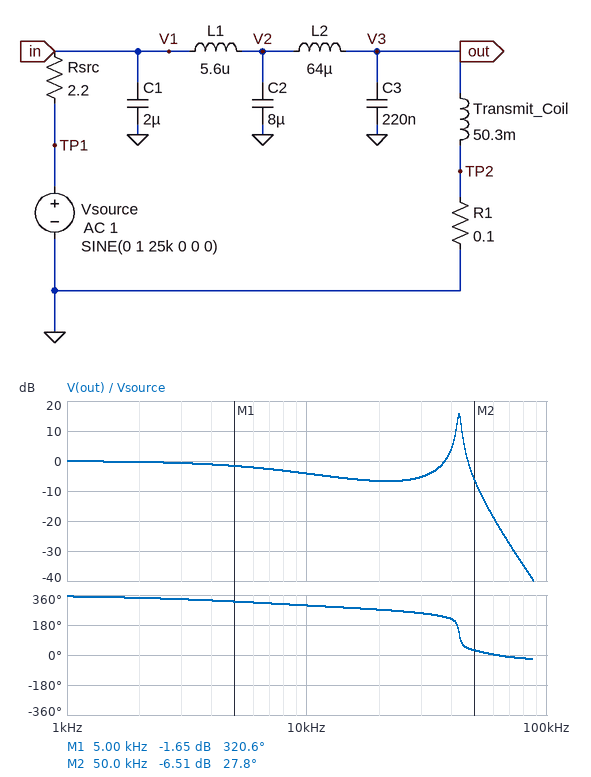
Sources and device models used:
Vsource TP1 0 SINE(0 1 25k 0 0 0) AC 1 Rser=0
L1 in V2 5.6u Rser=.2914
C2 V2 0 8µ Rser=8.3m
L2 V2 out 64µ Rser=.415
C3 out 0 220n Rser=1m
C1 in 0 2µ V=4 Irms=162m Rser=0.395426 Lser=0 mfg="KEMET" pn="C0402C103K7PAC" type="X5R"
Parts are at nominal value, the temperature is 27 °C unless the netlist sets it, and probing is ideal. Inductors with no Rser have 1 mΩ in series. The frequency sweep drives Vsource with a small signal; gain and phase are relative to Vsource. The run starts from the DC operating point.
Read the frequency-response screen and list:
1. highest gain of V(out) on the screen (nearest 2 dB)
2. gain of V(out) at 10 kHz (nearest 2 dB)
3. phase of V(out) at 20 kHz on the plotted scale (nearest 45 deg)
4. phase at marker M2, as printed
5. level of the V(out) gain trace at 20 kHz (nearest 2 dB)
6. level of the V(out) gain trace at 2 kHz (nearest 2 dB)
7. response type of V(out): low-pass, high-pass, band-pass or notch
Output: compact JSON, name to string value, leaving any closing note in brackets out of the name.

{"highest gain of V(out) on the screen": "16 dB", "gain of V(out) at 10 kHz": "-4 dB", "phase of V(out) at 20 kHz on the plotted scale": "270 deg", "phase at marker M2, as printed": "27.8 deg", "level of the V(out) gain trace at 20 kHz": "-6 dB", "level of the V(out) gain trace at 2 kHz": "0 dB", "response type of V(out): low-pass, high-pass, band-pass or notch": "band-pass"}
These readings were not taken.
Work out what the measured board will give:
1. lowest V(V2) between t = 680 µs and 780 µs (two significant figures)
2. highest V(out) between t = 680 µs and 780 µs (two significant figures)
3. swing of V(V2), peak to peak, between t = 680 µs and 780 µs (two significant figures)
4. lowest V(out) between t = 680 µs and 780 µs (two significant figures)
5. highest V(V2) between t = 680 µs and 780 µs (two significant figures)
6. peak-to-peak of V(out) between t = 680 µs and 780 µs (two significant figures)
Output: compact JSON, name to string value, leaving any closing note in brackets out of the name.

{"lowest V(V2) between t = 680 µs and 780 µs": "-310 mV", "highest V(out) between t = 680 µs and 780 µs": "480 mV", "swing of V(V2), peak to peak, between t = 680 µs and 780 µs": "620 mV", "lowest V(out) between t = 680 µs and 780 µs": "-480 mV", "highest V(V2) between t = 680 µs and 780 µs": "310 mV", "peak-to-peak of V(out) between t = 680 µs and 780 µs": "960 mV"}
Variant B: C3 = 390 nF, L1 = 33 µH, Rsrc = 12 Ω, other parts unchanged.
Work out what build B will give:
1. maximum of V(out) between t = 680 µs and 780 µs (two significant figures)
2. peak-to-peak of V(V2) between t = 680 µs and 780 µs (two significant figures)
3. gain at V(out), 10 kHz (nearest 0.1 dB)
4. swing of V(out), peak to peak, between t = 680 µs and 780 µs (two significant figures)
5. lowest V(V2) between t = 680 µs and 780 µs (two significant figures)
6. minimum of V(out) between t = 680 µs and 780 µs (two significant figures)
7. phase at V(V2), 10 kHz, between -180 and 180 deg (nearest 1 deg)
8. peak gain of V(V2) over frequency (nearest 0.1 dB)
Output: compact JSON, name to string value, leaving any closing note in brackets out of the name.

{"maximum of V(out) between t = 680 µs and 780 µs": "210 mV", "peak-to-peak of V(V2) between t = 680 µs and 780 µs": "160 mV", "gain at V(out), 10 kHz": "-15.2 dB", "swing of V(out), peak to peak, between t = 680 µs and 780 µs": "430 mV", "lowest V(V2) between t = 680 µs and 780 µs": "-82 mV", "minimum of V(out) between t = 680 µs and 780 µs": "-210 mV", "phase at V(V2), 10 kHz, between -180 and 180 deg": "-93 deg", "peak gain of V(V2) over frequency": "0 dB"}
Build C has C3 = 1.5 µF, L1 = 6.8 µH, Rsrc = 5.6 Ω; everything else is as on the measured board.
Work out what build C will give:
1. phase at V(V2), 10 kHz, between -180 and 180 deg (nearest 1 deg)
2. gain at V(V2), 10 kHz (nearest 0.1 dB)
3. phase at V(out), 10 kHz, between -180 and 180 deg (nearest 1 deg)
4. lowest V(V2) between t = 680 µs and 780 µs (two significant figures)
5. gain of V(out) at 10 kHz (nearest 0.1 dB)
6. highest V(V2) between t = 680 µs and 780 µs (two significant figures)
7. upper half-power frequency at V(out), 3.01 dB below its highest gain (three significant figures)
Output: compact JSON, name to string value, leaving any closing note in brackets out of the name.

{"phase at V(V2), 10 kHz, between -180 and 180 deg": "-81 deg", "gain at V(V2), 10 kHz": "-12.9 dB", "phase at V(out), 10 kHz, between -180 and 180 deg": "-85 deg", "lowest V(V2) between t = 680 µs and 780 µs": "-160 mV", "gain of V(out) at 10 kHz": "-8.8 dB", "highest V(V2) between t = 680 µs and 780 µs": "160 mV", "upper half-power frequency at V(out), 3.01 dB below its highest gain": "18.1 kHz"}
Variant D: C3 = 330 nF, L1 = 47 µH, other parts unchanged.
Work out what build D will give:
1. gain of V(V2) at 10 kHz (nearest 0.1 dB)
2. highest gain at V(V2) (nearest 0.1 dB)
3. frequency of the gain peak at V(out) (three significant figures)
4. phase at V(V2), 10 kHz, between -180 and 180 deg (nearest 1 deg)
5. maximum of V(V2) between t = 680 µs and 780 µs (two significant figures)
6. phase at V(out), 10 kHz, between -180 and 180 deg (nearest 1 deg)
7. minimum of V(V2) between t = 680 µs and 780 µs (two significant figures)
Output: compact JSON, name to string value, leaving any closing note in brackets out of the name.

{"gain of V(V2) at 10 kHz": "-2.3 dB", "highest gain at V(V2)": "0.4 dB", "frequency of the gain peak at V(out)": "35.4 kHz", "phase at V(V2), 10 kHz, between -180 and 180 deg": "-117 deg", "maximum of V(V2) between t = 680 µs and 780 µs": "95 mV", "phase at V(out), 10 kHz, between -180 and 180 deg": "-118 deg", "minimum of V(V2) between t = 680 µs and 780 µs": "-96 mV"}
